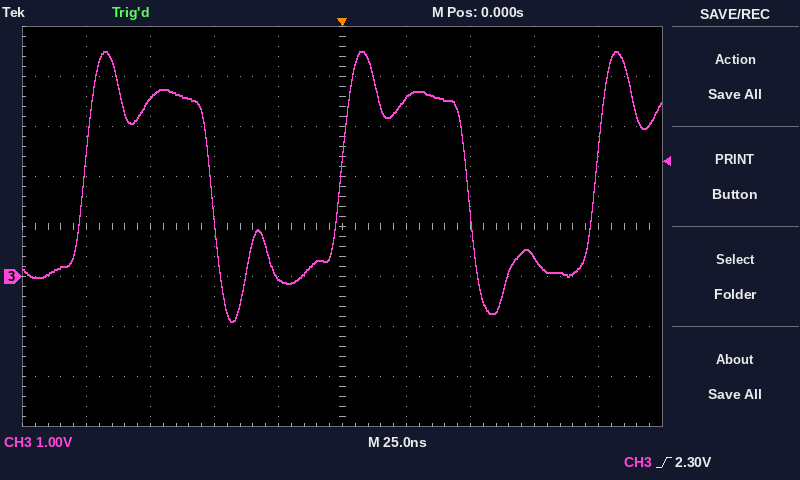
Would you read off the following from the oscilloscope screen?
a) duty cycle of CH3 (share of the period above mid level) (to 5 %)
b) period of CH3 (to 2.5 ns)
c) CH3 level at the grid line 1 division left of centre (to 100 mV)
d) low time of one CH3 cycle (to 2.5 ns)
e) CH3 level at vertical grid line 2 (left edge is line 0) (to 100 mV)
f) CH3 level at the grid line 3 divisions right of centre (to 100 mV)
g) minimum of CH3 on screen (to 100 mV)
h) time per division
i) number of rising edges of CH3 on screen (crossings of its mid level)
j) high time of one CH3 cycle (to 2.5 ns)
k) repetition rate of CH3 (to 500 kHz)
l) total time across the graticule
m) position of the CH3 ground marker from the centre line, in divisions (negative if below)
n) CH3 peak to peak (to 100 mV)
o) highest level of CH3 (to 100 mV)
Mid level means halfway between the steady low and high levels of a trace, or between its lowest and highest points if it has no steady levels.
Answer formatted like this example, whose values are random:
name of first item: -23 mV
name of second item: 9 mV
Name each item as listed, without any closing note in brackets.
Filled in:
duty cycle of CH3 (share of the period above mid level): 50 %
period of CH3: 100.0 ns
CH3 level at the grid line 1 division left of centre: 0.0 V
low time of one CH3 cycle: 50.0 ns
CH3 level at vertical grid line 2 (left edge is line 0): 3.6 V
CH3 level at the grid line 3 divisions right of centre: 400 mV
minimum of CH3 on screen: -900 mV
time per division: 25 ns
number of rising edges of CH3 on screen: 3
high time of one CH3 cycle: 50.0 ns
repetition rate of CH3: 10.0 MHz
total time across the graticule: 250 ns
position of the CH3 ground marker from the centre line, in divisions: -1.0 div
CH3 peak to peak: 5.4 V
highest level of CH3: 4.5 V
